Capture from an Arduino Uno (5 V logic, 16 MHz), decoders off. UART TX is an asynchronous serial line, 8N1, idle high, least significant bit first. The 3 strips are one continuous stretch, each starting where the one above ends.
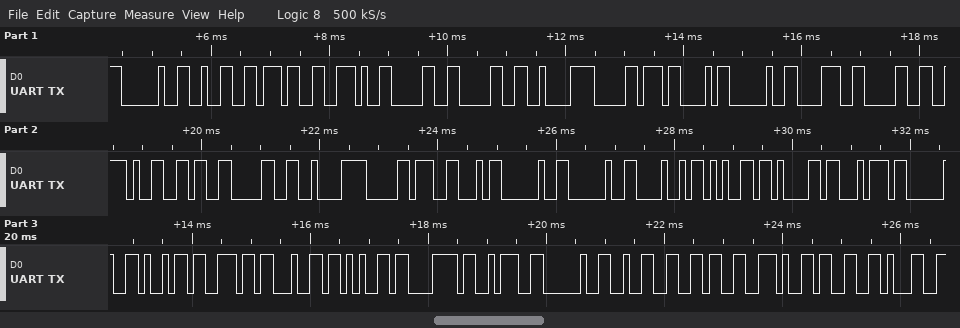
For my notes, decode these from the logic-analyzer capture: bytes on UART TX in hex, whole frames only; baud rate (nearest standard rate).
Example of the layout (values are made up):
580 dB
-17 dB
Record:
20 32 37 2E 30 30 C2 B0 43 20 38 30 2E 36 30 C2 B0 46 20 20 48 65 61 74 20 69 6E 64 65 78 3A 20 32 36 2E 33 31
9600 baud
